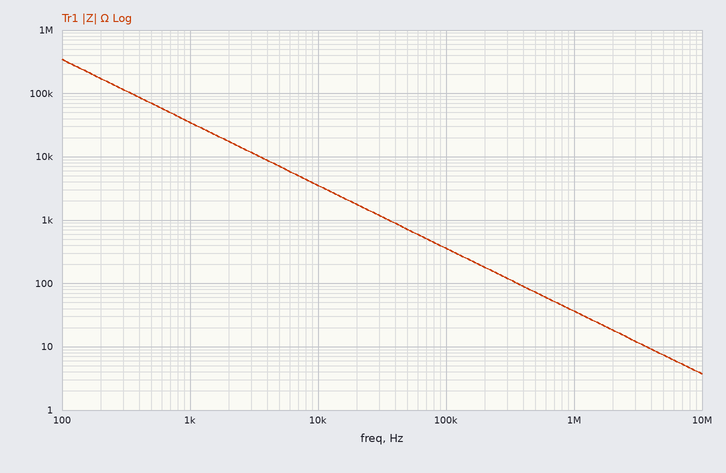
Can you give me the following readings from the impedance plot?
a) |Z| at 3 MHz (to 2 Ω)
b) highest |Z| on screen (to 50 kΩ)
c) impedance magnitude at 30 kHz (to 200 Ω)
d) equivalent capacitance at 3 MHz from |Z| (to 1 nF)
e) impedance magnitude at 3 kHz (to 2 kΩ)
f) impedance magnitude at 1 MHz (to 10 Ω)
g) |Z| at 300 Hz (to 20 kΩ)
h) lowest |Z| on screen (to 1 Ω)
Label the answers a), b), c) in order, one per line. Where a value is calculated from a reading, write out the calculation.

a) 12 Ω
b) 350 kΩ
c) 1.2 kΩ
d) C = 1/(2π × 3 MHz × 12 Ω) ≈ 4 nF
e) 12 kΩ
f) 40 Ω
g) 120 kΩ
h) 4 Ω
